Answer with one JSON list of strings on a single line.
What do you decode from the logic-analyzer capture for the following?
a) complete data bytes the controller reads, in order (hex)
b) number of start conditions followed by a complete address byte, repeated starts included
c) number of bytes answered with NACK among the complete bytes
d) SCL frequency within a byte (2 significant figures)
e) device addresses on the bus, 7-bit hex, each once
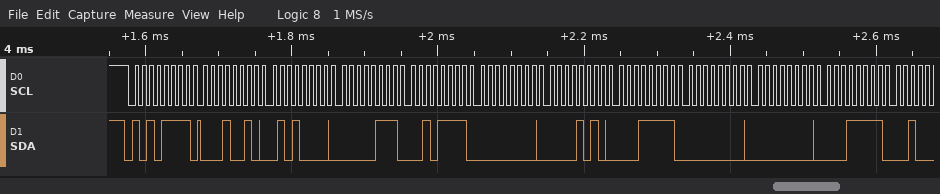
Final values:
["12 50 07 2F 00 0A 1F 00 00 1F", "1", "0", "100 kHz", "0x57"]
